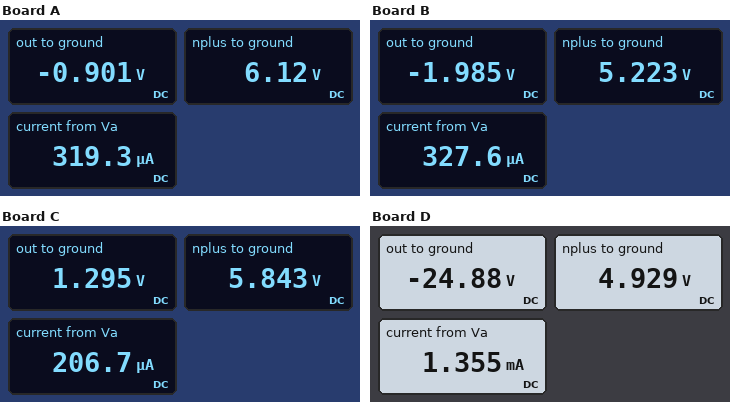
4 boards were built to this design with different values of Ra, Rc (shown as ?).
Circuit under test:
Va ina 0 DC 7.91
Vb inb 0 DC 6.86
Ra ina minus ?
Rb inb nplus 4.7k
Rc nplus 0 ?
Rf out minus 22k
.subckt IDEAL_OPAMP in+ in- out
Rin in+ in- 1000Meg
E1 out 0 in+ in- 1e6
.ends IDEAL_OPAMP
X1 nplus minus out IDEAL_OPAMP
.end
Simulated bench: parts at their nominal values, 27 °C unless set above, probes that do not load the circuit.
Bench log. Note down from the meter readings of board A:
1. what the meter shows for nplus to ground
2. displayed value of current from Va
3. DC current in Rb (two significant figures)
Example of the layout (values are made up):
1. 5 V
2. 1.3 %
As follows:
1. 6.12 V
2. 319.3 µA
3. 160 µA
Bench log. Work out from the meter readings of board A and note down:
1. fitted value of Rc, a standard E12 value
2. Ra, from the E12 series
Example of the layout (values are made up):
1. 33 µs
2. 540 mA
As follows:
1. 39 kΩ
2. 5.6 kΩ
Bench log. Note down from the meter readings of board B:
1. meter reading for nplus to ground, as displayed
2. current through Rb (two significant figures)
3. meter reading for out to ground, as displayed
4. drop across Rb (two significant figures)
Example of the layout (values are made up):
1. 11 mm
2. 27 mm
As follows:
1. 5.223 V
2. 350 µA
3. -1.985 V
4. 1.6 V
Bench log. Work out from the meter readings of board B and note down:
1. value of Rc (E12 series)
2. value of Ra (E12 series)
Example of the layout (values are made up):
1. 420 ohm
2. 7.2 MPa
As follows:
1. 15 kΩ
2. 8.2 kΩ
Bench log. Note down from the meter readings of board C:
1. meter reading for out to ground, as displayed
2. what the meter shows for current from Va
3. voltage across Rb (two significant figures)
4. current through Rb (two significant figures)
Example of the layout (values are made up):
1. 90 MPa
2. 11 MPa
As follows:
1. 1.295 V
2. 206.7 µA
3. 1.0 V
4. 220 µA
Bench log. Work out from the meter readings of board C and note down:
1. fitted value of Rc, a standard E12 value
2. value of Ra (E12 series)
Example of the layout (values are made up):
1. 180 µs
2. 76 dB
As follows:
1. 27 kΩ
2. 10 kΩ
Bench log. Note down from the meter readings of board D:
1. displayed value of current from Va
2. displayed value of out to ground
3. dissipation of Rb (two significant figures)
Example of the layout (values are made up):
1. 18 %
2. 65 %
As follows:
1. 1.355 mA
2. -24.88 V
3. 790 µW
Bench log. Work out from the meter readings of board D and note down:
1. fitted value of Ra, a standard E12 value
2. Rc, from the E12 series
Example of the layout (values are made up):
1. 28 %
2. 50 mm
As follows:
1. 2.2 kΩ
2. 12 kΩ
